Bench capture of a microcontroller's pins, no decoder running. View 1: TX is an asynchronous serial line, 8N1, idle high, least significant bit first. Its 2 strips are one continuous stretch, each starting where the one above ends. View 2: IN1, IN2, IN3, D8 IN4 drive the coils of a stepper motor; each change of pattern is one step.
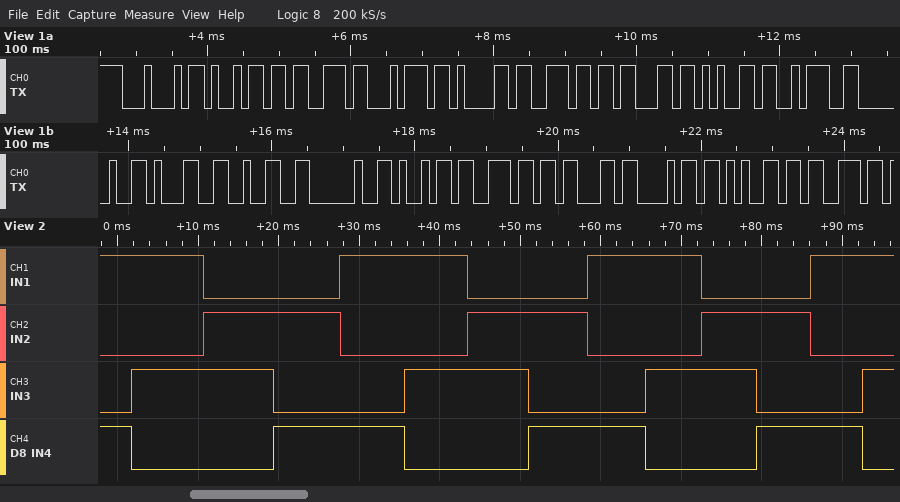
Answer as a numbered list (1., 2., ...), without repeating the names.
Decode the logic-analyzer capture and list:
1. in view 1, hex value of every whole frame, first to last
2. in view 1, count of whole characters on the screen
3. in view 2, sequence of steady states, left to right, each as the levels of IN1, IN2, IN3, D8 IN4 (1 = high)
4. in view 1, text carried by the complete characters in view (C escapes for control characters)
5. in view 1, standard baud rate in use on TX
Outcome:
1. 44 69 73 74 61 6E 63 65 3A 20 31 32 20 69 6E 63 68 65 73
2. 19
3. 1001 1010 0110 0101 1001 1010 0110 0101 1001 1010 0110 0101 1001 1010
4. "Distance: 12 inches"
5. 9600 baud
